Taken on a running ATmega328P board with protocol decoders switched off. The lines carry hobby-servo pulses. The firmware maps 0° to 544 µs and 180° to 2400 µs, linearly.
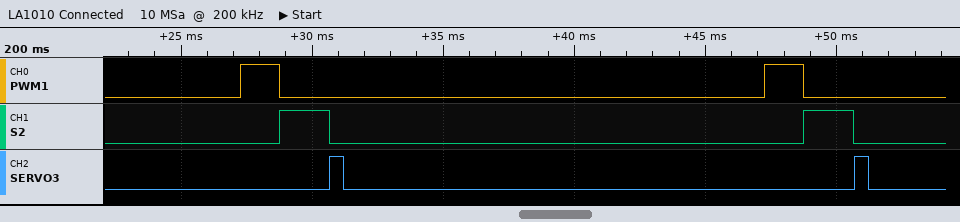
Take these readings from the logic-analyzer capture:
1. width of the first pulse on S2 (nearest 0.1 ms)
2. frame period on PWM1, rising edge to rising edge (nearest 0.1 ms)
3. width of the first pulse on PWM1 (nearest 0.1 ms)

1.9 ms
20.0 ms
1.5 ms
